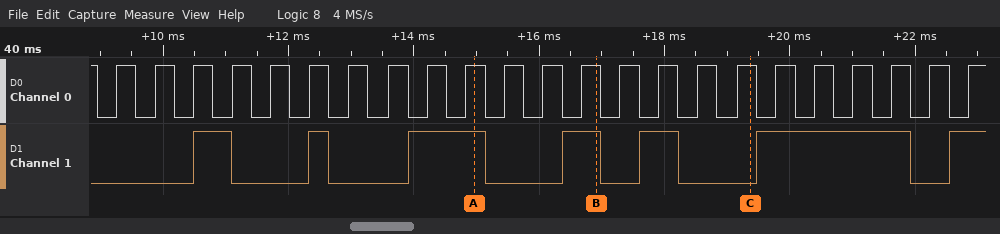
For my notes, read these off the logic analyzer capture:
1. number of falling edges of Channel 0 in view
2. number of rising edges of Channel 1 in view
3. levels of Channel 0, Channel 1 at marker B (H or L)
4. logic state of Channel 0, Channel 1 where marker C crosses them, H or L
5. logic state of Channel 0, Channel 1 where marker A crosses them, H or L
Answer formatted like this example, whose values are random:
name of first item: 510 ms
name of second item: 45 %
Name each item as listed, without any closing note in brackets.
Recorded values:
number of falling edges of Channel 0 in view: 23
number of rising edges of Channel 1 in view: 7
levels of Channel 0, Channel 1 at marker B: Channel 0=H, Channel 1=H
logic state of Channel 0, Channel 1 where marker C crosses them, H or L: Channel 0=H, Channel 1=L
logic state of Channel 0, Channel 1 where marker A crosses them, H or L: Channel 0=H, Channel 1=H
